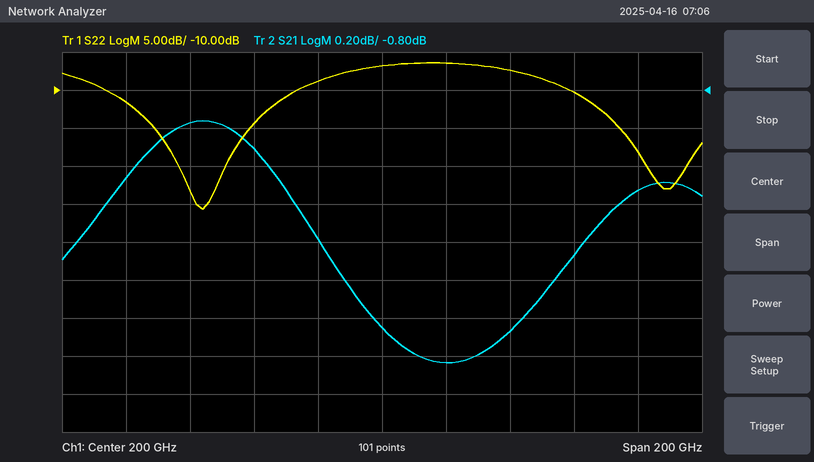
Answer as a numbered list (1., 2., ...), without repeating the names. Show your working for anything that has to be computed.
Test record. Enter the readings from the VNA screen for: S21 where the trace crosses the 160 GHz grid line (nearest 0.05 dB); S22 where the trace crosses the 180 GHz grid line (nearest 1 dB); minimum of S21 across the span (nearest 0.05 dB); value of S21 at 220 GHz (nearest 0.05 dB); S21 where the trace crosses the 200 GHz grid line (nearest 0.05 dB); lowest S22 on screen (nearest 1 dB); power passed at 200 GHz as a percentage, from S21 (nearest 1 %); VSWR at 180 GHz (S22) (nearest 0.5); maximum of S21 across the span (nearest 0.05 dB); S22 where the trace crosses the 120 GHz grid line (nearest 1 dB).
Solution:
1. -1.10 dB
2. -9 dB
3. -2.25 dB
4. -2.25 dB
5. -2.05 dB
6. -26 dB
7. 10^(-2.05/10) ≈ 62 %
8. |Γ| = 10^(-9/20) = 0.3548; VSWR = (1 + 0.3548)/(1 − 0.3548) ≈ 2.10, so 2.0 to the nearest 0.5
9. -0.95 dB
10. -12 dB
